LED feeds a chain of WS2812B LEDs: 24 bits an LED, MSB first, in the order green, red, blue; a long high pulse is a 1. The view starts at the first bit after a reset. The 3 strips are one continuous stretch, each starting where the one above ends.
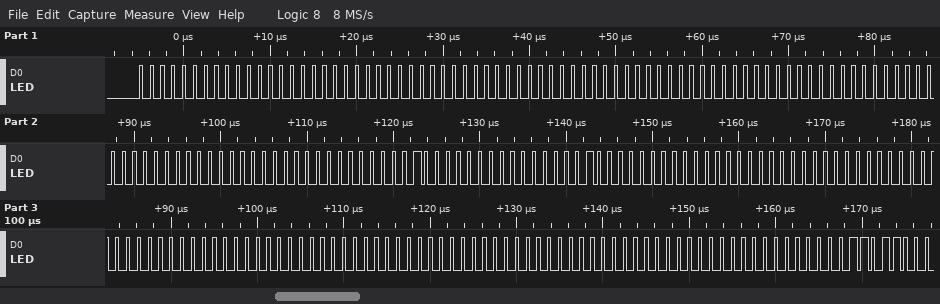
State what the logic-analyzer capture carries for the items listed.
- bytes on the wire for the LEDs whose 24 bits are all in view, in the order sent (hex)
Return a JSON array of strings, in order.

["00 00 00 00 00 00 00 00 00 00 00 00 02 00 02 00 00 00 00 00 00 00 00 00 00 00 00"]
